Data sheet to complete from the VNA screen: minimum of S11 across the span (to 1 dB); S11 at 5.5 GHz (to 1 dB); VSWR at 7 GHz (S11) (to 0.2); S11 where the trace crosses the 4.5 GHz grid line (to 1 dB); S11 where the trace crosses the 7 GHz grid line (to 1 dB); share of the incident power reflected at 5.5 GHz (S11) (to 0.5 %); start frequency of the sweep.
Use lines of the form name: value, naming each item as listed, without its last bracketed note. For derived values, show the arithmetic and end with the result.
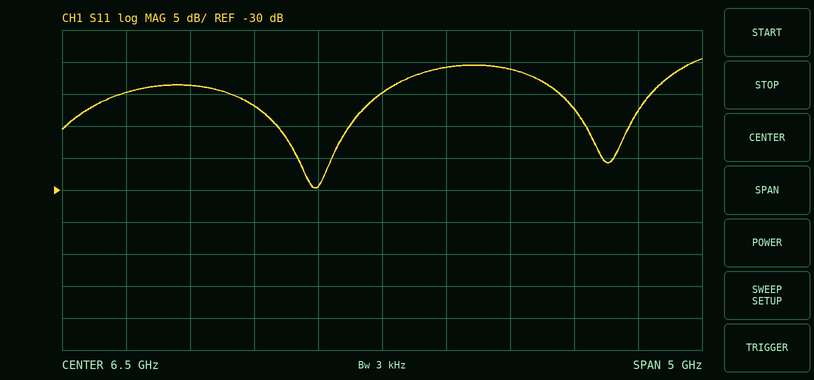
minimum of S11 across the span: -30 dB
S11 at 5.5 GHz: -17 dB
VSWR at 7 GHz (S11): |Γ| = 10^(-11/20) = 0.2818; VSWR = (1 + 0.2818)/(1 − 0.2818) ≈ 1.8
S11 where the trace crosses the 4.5 GHz grid line: -15 dB
S11 where the trace crosses the 7 GHz grid line: -11 dB
share of the incident power reflected at 5.5 GHz (S11): 10^(-17/10) ≈ 2.0 %
start frequency of the sweep: 4 GHz
